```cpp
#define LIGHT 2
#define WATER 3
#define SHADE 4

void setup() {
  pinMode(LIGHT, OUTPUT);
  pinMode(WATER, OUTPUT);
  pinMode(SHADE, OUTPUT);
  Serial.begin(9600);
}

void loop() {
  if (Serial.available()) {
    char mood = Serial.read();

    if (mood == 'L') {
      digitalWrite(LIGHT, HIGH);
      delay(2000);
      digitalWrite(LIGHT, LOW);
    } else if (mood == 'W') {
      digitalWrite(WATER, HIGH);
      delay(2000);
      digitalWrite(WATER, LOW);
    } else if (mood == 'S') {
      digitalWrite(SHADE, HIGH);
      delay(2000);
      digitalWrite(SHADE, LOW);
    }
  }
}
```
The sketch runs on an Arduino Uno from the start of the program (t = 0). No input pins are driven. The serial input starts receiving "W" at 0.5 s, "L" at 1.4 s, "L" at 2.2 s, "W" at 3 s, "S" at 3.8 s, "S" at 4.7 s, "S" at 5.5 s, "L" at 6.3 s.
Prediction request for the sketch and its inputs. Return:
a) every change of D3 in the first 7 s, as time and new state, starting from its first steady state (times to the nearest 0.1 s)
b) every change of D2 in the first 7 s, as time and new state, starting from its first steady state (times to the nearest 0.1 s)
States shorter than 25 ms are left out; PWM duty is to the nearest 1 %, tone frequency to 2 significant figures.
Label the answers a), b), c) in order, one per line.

a) 0 s low; 0.5 s high; 2.5 s low; 6.5 s high
b) 0 s low; 2.5 s high; 6.5 s low
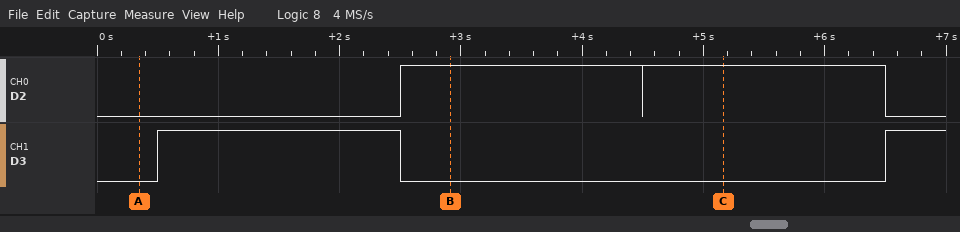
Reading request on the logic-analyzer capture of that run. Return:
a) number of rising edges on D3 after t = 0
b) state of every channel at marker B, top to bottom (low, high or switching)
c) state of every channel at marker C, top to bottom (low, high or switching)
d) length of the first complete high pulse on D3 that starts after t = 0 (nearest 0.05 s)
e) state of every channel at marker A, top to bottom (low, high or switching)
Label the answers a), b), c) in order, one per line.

a) 2
b) D2 high, D3 low
c) D2 high, D3 low
d) 2.00 s
e) D2 low, D3 low
